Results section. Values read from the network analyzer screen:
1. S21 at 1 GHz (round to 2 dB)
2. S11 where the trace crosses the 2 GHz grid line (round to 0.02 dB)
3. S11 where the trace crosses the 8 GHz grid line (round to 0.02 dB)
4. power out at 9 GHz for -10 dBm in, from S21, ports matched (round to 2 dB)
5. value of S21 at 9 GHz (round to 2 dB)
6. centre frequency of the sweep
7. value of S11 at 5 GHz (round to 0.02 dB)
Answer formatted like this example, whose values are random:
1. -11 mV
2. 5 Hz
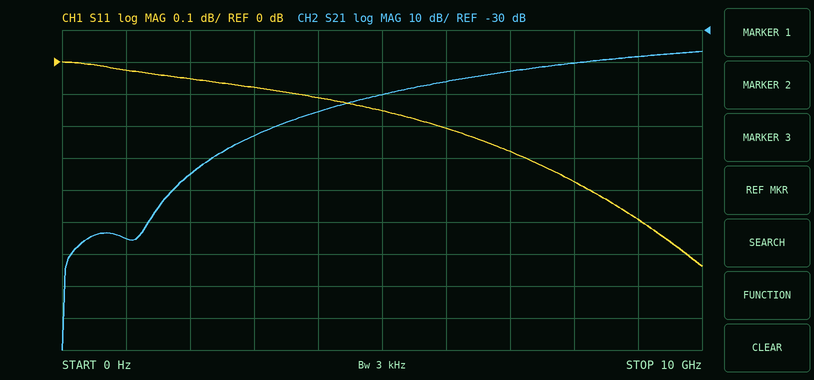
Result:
1. -96 dB
2. -0.06 dB
3. -0.38 dB
4. -48 dBm
5. -38 dB
6. 5 GHz
7. -0.16 dB
